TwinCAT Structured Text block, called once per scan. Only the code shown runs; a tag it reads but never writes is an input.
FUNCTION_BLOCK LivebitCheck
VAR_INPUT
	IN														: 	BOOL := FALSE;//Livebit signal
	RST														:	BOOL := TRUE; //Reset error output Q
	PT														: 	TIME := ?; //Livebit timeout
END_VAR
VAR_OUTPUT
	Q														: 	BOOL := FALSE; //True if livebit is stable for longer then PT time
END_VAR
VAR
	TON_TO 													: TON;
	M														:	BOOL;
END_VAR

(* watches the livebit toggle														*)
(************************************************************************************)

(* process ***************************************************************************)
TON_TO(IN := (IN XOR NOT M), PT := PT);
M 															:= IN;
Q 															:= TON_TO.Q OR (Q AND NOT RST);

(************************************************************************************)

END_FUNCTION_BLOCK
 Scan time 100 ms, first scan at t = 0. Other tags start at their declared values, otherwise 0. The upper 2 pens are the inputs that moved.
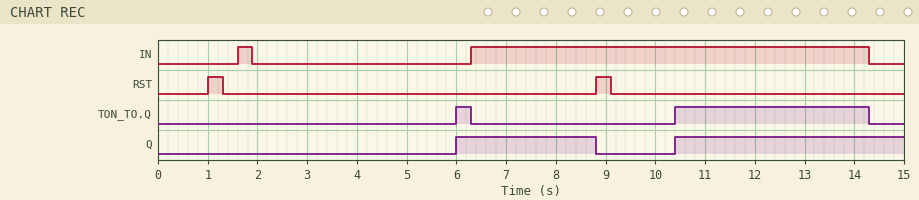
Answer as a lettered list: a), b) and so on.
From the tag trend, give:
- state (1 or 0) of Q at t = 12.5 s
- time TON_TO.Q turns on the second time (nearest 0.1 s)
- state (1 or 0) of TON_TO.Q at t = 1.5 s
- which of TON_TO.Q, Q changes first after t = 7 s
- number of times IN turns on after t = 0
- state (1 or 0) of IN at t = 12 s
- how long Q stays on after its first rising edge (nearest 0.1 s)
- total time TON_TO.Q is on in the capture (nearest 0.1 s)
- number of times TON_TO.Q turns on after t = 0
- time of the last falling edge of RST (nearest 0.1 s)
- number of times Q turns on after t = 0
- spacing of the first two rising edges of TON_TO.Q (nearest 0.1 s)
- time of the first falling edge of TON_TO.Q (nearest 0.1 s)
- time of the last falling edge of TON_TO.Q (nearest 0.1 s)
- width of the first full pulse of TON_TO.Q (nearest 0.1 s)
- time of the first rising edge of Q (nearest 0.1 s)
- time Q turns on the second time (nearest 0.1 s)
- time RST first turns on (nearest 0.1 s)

a) 1
b) 10.4 s
c) 0
d) Q
e) 2
f) 1
g) 2.8 s
h) 4.2 s
i) 2
j) 9.1 s
k) 2
l) 4.4 s
m) 6.3 s
n) 14.3 s
o) 0.3 s
p) 6.0 s
q) 10.4 s
r) 1.0 s
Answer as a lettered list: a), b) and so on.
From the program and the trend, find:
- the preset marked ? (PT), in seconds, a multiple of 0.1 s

a) 4.0 s
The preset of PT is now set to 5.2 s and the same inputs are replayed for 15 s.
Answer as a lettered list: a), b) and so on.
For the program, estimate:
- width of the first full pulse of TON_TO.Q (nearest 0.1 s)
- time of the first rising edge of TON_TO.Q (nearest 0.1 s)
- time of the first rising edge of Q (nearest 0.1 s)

a) 2.7 s
b) 11.6 s
c) 11.6 s
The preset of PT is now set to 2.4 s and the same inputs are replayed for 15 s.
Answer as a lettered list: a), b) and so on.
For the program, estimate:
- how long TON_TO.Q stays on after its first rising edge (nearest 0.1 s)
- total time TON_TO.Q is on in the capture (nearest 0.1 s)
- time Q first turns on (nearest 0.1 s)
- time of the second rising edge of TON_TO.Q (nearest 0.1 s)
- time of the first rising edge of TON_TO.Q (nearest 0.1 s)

a) 1.9 s
b) 7.4 s
c) 4.4 s
d) 8.8 s
e) 4.4 s
